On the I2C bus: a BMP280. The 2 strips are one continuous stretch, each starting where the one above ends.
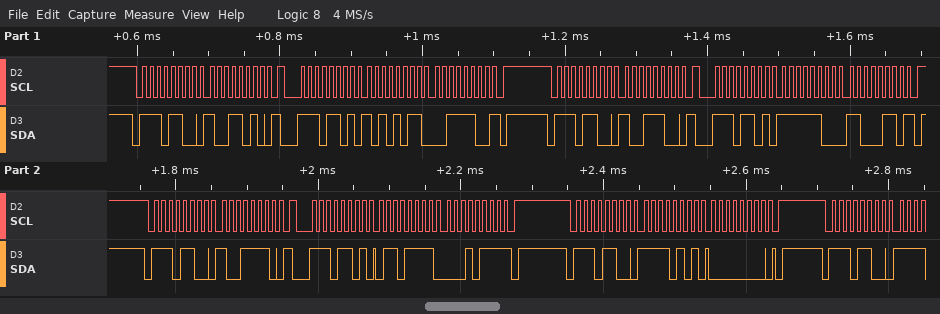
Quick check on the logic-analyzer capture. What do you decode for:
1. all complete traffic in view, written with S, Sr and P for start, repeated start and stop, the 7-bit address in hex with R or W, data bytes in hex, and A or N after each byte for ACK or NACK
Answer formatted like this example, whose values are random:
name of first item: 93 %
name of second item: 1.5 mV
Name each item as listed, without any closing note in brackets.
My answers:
all complete traffic in view, written with S, Sr and P for start, repeated start and stop, the 7-bit address in hex with R or W, data bytes in hex, and A or N after each byte for ACK or NACK: S 76W A 9A A Sr 76R A AB A 3C N P S 76W A 9C A Sr 76R A FC A C6 N P S 76W A 9E A Sr 76R A 6F A 17 N P S 76W A F5 A 00 A P S 76W A
